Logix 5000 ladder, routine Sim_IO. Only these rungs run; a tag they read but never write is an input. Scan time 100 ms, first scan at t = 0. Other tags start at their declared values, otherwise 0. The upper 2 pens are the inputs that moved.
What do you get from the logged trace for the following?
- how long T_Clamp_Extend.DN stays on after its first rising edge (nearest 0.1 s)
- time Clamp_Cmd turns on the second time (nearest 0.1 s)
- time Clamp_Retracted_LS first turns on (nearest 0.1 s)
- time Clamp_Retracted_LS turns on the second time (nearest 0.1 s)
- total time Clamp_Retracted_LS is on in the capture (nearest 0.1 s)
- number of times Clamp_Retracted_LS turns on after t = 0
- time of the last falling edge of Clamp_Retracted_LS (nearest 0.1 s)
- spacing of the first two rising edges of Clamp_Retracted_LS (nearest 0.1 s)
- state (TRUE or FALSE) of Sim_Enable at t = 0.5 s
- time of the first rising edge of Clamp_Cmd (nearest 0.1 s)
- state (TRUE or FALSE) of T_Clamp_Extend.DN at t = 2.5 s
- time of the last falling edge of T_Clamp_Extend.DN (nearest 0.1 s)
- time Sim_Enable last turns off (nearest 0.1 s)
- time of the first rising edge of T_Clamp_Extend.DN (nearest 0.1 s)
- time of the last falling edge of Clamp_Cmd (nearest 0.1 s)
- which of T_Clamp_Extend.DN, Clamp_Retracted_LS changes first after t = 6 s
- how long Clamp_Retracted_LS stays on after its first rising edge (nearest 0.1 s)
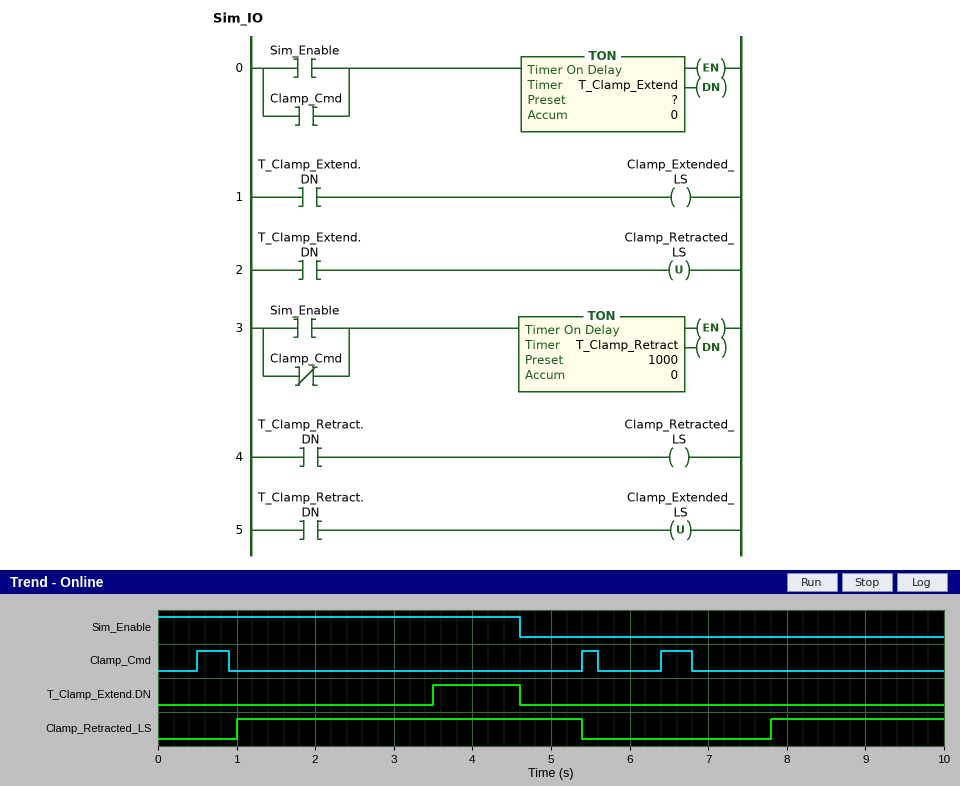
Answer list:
1.1 s
5.4 s
1.0 s
7.8 s
6.6 s
2
5.4 s
6.8 s
TRUE
0.5 s
FALSE
4.6 s
4.6 s
3.5 s
6.8 s
Clamp_Retracted_LS
4.4 s
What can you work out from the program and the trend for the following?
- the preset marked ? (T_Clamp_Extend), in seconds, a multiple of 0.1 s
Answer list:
3.5 s
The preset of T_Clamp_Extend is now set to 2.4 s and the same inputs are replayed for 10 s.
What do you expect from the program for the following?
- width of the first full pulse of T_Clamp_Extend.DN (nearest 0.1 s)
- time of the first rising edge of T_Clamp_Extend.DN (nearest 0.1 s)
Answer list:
2.2 s
2.4 s
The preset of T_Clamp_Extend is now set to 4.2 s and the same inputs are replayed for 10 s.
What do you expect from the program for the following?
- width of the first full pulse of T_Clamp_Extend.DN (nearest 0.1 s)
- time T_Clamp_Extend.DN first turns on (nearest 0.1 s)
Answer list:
0.4 s
4.2 s
